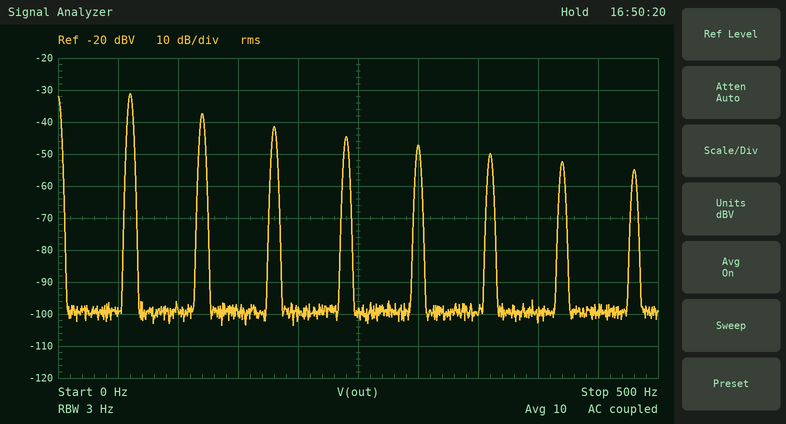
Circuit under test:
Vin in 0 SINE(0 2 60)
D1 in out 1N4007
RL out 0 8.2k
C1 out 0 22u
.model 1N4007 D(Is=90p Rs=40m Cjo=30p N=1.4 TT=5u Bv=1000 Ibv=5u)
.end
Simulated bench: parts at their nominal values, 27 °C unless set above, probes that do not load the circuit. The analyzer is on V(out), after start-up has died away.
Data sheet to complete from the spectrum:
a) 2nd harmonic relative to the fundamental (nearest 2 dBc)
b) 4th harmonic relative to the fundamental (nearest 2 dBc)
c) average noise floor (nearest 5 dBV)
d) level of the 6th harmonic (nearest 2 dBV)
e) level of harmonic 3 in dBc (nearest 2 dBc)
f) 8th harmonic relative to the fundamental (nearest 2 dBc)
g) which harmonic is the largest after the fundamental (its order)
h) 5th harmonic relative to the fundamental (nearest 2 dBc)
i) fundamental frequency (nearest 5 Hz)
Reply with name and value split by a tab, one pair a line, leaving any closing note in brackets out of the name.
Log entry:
2nd harmonic relative to the fundamental	-6 dBc
4th harmonic relative to the fundamental	-14 dBc
average noise floor	-100 dBV
level of the 6th harmonic	-50 dBV
level of harmonic 3 in dBc	-10 dBc
8th harmonic relative to the fundamental	-24 dBc
which harmonic is the largest after the fundamental	2
5th harmonic relative to the fundamental	-16 dBc
fundamental frequency	60 Hz
